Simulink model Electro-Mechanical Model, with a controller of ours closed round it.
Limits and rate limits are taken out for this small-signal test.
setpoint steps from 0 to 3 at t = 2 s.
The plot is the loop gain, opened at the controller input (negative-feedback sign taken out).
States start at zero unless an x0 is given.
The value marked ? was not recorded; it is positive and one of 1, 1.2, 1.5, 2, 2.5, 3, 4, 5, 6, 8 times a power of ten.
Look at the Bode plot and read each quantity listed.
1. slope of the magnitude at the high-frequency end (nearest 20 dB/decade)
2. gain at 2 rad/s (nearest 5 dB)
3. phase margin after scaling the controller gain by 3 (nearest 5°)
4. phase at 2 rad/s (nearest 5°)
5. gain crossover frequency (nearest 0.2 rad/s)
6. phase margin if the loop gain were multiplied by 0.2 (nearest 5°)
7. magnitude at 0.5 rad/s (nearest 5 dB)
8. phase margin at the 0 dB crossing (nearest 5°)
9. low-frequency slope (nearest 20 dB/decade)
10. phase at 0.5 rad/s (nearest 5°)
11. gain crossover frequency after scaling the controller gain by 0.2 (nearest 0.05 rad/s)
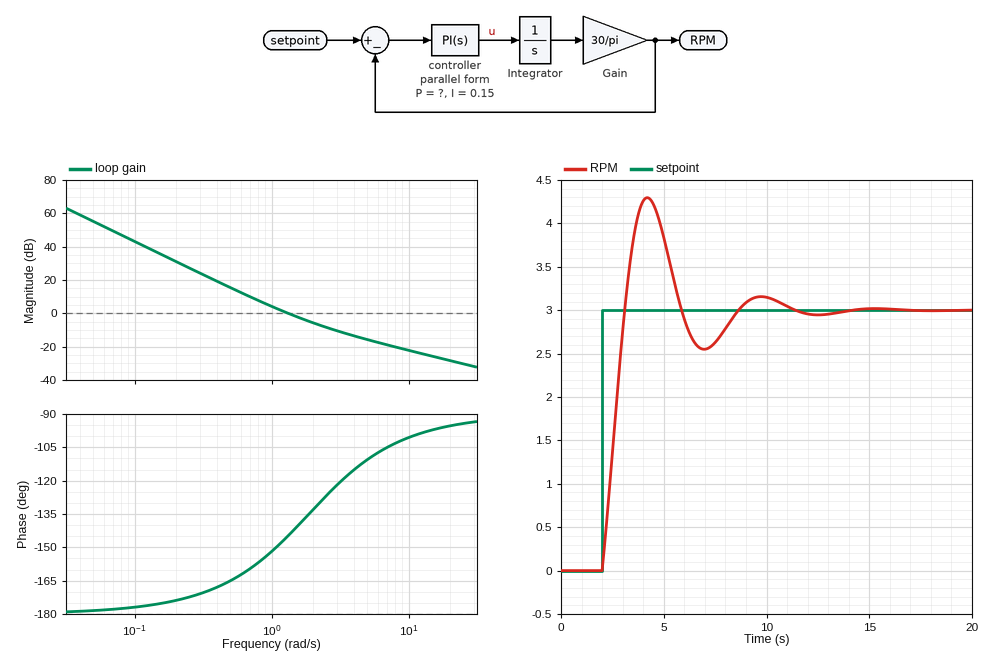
-20 dB/decade
-5 dB
55°
-135°
1.4 rad/s
15°
15 dB
35°
-40 dB/decade
-165°
0.55 rad/s
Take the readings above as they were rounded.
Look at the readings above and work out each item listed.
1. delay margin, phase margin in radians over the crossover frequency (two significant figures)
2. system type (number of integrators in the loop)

0.44 s
2
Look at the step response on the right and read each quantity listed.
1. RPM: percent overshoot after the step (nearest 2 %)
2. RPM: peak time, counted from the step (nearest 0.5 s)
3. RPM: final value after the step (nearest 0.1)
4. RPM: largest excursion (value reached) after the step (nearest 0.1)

44 %
2.0 s
3.0
4.3
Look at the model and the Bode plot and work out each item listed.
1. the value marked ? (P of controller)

0.08
